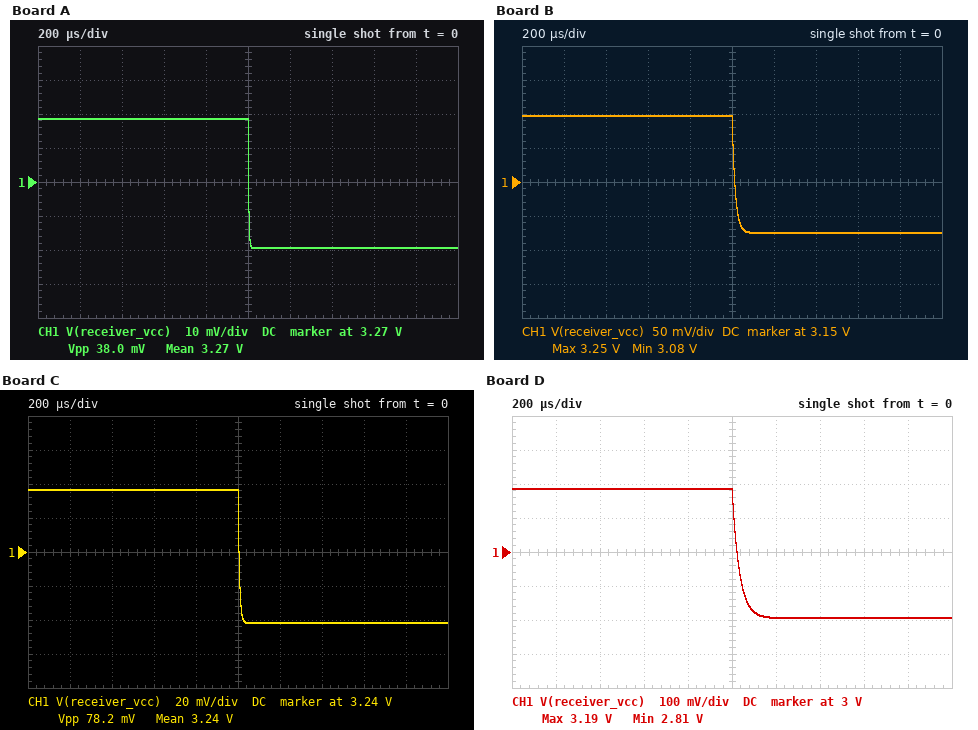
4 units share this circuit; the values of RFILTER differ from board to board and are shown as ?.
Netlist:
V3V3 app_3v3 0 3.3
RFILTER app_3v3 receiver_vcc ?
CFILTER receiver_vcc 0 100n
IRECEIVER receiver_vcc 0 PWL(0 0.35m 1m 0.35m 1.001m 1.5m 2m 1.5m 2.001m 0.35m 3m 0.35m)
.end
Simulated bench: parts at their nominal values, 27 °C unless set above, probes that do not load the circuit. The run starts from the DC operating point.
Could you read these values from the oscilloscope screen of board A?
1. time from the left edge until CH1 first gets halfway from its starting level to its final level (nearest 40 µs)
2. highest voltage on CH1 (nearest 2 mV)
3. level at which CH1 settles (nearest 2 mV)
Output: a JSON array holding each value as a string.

["1.00 ms", "3.288 V", "3.250 V"]
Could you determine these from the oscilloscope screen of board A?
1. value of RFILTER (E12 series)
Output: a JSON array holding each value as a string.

["33 Ω"]
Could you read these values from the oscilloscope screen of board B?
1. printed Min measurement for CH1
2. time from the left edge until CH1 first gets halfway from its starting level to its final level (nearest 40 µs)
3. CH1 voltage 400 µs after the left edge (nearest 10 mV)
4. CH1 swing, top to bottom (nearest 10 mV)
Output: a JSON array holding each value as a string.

["3.08 V", "1.00 ms", "3.25 V", "170 mV"]
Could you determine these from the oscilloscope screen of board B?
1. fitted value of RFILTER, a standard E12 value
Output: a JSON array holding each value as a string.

["150 Ω"]
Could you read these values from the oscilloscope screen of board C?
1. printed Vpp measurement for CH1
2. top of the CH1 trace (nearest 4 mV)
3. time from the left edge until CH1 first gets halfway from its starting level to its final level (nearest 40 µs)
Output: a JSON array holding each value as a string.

["78.2 mV", "3.276 V", "1.00 ms"]
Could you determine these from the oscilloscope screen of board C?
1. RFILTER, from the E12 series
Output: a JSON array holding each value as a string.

["68 Ω"]
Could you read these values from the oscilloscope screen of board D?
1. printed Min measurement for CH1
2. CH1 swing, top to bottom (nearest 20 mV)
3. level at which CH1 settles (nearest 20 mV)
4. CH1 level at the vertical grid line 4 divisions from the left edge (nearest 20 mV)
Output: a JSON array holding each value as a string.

["2.81 V", "380 mV", "2.80 V", "3.18 V"]
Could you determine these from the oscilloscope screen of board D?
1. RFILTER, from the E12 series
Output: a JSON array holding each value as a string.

["330 Ω"]
